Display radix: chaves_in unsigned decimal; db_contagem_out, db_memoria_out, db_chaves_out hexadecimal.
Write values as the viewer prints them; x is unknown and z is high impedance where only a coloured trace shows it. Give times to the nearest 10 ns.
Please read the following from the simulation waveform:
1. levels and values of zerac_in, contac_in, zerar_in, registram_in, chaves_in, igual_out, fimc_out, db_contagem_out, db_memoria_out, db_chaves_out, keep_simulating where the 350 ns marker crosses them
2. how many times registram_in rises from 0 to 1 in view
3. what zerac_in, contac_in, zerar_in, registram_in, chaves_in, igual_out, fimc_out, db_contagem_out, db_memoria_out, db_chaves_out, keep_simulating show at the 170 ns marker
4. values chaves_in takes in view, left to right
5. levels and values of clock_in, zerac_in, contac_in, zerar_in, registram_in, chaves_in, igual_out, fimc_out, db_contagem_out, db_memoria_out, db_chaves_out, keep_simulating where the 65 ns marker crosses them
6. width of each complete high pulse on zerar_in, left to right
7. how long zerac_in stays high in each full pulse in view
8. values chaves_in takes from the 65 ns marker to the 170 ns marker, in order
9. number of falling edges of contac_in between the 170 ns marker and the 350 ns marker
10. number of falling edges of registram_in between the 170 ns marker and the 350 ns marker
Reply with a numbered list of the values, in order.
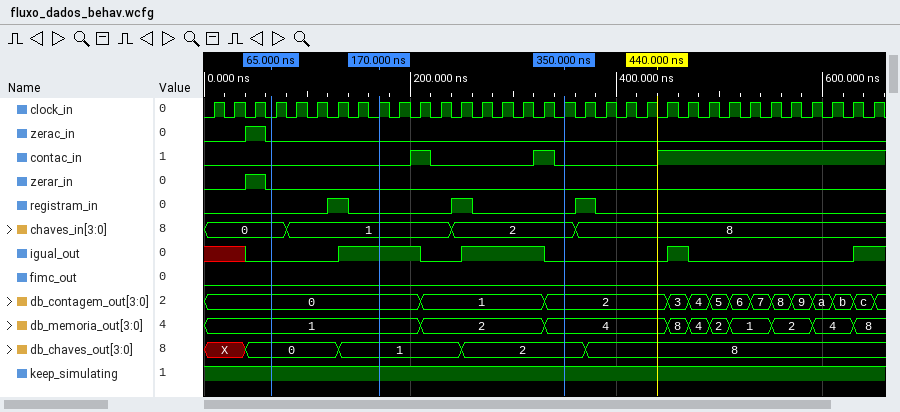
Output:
1. zerac_in=0, contac_in=0, zerar_in=0, registram_in=0, chaves_in=2, igual_out=0, fimc_out=0, db_contagem_out=2, db_memoria_out=4, db_chaves_out=2, keep_simulating=1
2. 3
3. zerac_in=0, contac_in=0, zerar_in=0, registram_in=0, chaves_in=1, igual_out=1, fimc_out=0, db_contagem_out=0, db_memoria_out=1, db_chaves_out=1, keep_simulating=1
4. 0, 1, 2, 8
5. clock_in=0, zerac_in=0, contac_in=0, zerar_in=0, registram_in=0, chaves_in=0, igual_out=0, fimc_out=0, db_contagem_out=0, db_memoria_out=1, db_chaves_out=0, keep_simulating=1
6. 20 ns
7. 20 ns
8. 0, 1
9. 2
10. 1
